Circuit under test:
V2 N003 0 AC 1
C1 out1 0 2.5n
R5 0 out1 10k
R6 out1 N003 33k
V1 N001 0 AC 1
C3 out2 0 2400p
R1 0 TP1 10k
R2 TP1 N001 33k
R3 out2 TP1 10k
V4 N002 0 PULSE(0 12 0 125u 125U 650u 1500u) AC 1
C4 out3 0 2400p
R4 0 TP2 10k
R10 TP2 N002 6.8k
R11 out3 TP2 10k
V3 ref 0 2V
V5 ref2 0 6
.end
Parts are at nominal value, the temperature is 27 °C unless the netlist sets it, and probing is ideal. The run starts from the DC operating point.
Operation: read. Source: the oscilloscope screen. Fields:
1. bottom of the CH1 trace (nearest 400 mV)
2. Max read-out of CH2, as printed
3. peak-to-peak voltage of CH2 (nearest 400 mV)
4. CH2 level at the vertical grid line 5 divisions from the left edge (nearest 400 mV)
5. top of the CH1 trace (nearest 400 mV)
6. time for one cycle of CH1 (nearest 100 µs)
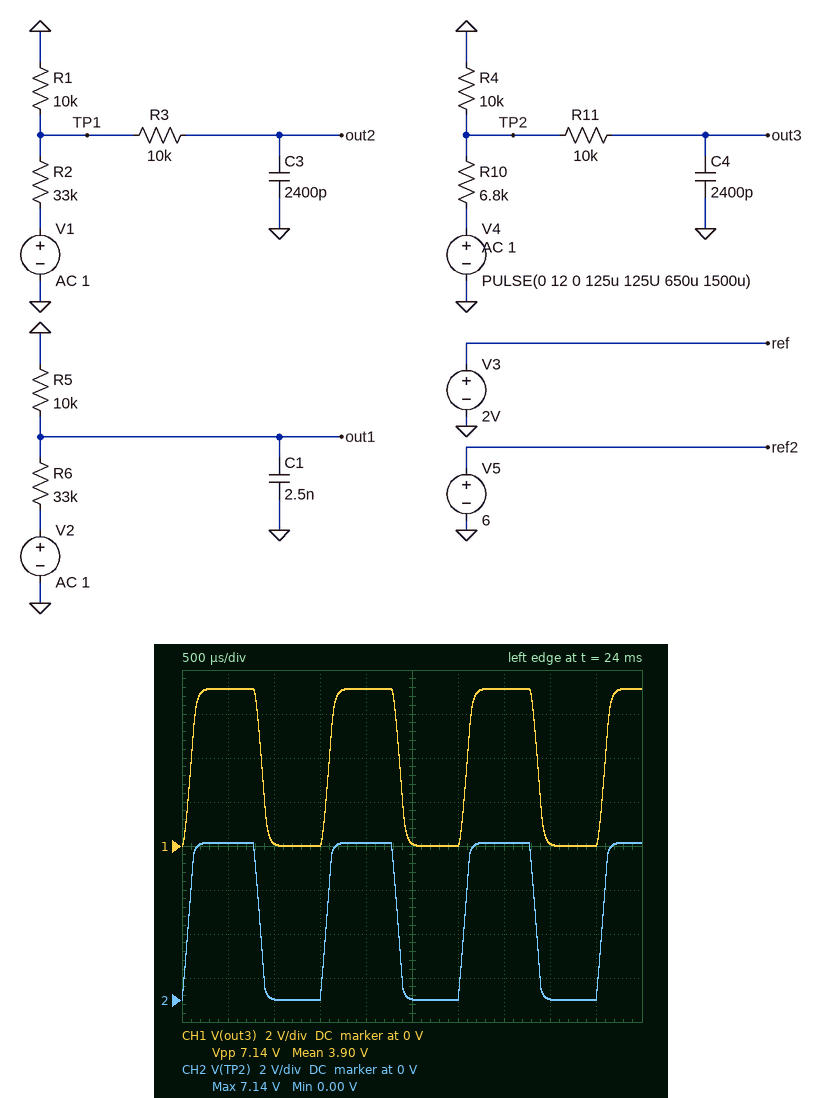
0 V
7.14 V
7.2 V
0 V
7.2 V
1.5 ms
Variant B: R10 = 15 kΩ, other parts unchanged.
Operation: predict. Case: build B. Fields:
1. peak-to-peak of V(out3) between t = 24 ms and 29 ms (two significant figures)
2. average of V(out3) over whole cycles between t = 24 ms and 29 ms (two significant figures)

4.8 V
2.5 V
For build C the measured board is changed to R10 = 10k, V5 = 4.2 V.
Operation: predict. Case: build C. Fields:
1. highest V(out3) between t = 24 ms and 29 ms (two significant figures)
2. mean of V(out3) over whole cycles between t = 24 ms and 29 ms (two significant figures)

6.0 V
3.1 V
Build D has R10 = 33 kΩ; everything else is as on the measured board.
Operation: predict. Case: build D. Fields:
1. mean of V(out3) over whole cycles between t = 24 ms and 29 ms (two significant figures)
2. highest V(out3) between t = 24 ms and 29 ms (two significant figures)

1.4 V
2.8 V
